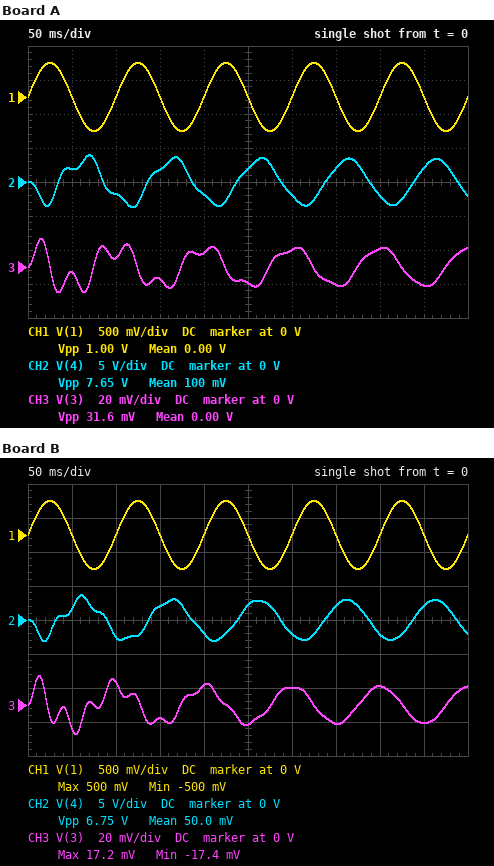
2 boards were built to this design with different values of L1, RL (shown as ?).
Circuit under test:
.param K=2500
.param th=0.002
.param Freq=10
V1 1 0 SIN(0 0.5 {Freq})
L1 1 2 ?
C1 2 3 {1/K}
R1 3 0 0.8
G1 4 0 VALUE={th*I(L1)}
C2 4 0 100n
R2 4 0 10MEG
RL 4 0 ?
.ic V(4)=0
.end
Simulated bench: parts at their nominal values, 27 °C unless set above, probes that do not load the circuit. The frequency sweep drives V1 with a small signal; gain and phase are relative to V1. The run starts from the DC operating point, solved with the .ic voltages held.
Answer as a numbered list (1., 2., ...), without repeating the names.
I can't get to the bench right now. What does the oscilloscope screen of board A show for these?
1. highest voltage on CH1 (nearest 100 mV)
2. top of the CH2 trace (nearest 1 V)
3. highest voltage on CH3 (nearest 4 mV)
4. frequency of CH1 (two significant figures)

1. 500 mV
2. 4 V
3. 16 mV
4. 10 Hz
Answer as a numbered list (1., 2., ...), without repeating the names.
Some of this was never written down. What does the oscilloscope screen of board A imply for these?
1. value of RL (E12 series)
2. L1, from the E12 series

1. 180 kΩ
2. 68 mH
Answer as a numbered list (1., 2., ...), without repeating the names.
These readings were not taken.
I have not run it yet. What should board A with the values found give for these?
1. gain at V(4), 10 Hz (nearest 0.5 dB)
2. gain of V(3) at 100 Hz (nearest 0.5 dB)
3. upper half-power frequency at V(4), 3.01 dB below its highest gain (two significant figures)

1. 16.5 dB
2. -33.5 dB
3. 31 Hz
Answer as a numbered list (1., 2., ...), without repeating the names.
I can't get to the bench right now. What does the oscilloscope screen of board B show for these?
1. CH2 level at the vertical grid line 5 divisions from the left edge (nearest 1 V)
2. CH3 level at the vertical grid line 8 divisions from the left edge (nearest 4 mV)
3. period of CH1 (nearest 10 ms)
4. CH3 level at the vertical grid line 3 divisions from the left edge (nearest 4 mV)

1. 2 V
2. 12 mV
3. 100 ms
4. -8 mV
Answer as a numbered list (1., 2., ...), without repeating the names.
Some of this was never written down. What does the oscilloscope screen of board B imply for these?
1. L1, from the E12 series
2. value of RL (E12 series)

1. 47 mH
2. 150 kΩ
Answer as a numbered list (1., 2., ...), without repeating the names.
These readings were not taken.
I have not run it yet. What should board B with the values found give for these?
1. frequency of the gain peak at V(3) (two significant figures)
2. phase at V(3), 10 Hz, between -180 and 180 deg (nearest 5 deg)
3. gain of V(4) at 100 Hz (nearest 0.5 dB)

1. 37 Hz
2. 90 deg
3. 2.0 dB
